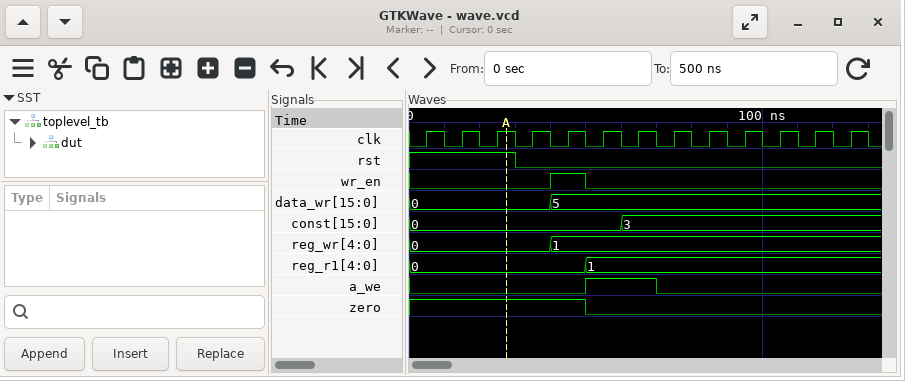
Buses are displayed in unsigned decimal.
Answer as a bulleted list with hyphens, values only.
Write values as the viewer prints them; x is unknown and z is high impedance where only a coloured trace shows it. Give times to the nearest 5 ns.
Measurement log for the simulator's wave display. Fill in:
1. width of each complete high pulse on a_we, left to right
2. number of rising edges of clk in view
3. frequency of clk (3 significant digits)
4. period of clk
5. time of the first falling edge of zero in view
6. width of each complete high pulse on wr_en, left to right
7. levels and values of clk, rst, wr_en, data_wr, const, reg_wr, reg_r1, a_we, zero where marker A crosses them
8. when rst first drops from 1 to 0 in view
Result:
- 20 ns
- 13
- 100 MHz
- 10 ns
- 50 ns
- 10 ns
- clk=1, rst=1, wr_en=0, data_wr=0, const=0, reg_wr=0, reg_r1=0, a_we=0, zero=1
- 30 ns
